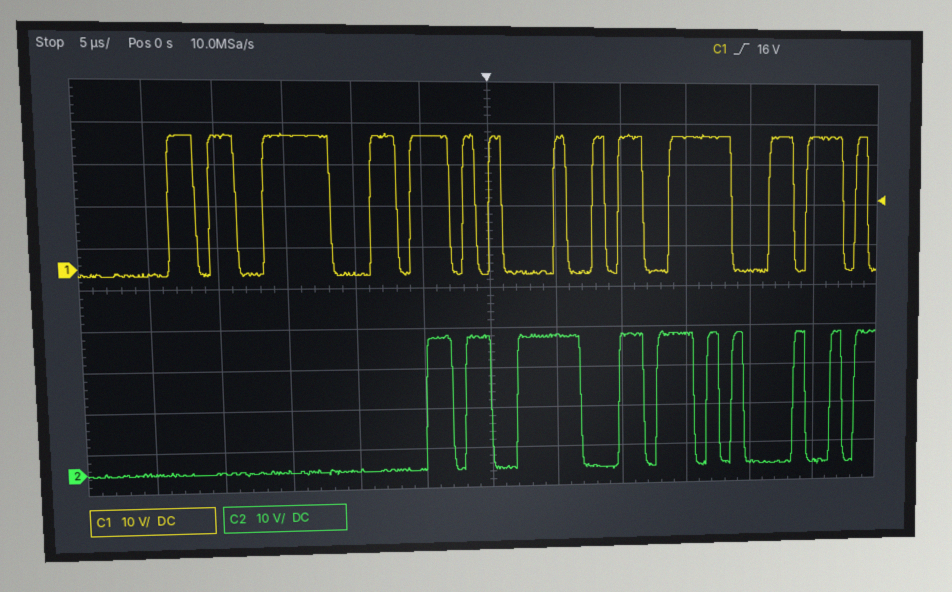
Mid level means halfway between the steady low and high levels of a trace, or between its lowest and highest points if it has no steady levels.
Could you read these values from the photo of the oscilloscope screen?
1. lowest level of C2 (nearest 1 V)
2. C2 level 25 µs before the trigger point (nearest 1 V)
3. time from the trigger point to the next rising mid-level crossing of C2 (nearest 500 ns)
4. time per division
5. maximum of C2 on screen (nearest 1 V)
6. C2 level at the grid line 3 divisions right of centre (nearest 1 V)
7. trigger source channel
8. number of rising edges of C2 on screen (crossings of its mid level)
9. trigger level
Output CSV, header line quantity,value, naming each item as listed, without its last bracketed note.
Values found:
quantity,value
lowest level of C2,-1 V
C2 level 25 µs before the trigger point,0 V
time from the trigger point to the next rising mid-level crossing of C2,2.0 µs
time per division,5 µs
maximum of C2 on screen,34 V
C2 level at the grid line 3 divisions right of centre,33 V
trigger source channel,C1
number of rising edges of C2 on screen,10
trigger level,16 V
